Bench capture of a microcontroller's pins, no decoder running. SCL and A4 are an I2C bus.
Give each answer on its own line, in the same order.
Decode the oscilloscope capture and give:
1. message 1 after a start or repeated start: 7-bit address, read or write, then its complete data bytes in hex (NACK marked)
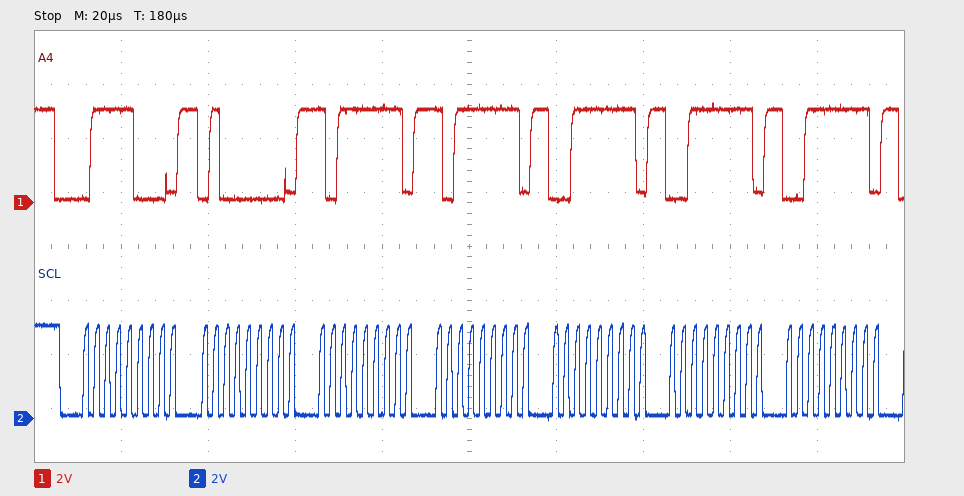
0x3C write: 40 BF BF 3F 3F 3F
